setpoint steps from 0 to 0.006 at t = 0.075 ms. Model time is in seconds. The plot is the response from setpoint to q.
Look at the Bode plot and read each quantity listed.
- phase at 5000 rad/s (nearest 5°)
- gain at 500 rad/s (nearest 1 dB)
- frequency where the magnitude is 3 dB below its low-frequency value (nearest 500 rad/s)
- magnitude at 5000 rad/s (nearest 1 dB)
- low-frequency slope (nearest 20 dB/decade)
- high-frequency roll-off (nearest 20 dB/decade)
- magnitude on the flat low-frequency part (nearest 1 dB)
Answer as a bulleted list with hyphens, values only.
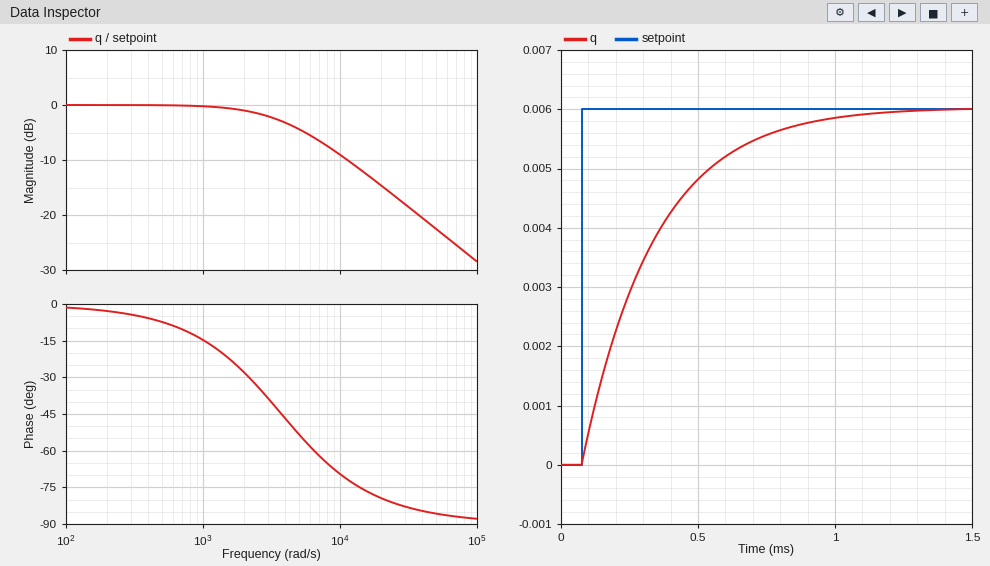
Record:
- -55°
- 0 dB
- 4000 rad/s
- -4 dB
- 0 dB/decade
- -20 dB/decade
- 0 dB
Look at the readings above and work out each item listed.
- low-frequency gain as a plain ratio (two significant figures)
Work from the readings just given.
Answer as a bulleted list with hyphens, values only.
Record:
- 1.0
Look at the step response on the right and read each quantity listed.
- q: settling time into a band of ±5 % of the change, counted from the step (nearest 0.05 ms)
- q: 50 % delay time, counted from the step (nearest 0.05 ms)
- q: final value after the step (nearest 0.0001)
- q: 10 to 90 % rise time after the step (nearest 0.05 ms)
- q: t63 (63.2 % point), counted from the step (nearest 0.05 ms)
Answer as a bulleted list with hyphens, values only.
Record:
- 0.75 ms
- 0.20 ms
- 0.0060
- 0.55 ms
- 0.25 ms
